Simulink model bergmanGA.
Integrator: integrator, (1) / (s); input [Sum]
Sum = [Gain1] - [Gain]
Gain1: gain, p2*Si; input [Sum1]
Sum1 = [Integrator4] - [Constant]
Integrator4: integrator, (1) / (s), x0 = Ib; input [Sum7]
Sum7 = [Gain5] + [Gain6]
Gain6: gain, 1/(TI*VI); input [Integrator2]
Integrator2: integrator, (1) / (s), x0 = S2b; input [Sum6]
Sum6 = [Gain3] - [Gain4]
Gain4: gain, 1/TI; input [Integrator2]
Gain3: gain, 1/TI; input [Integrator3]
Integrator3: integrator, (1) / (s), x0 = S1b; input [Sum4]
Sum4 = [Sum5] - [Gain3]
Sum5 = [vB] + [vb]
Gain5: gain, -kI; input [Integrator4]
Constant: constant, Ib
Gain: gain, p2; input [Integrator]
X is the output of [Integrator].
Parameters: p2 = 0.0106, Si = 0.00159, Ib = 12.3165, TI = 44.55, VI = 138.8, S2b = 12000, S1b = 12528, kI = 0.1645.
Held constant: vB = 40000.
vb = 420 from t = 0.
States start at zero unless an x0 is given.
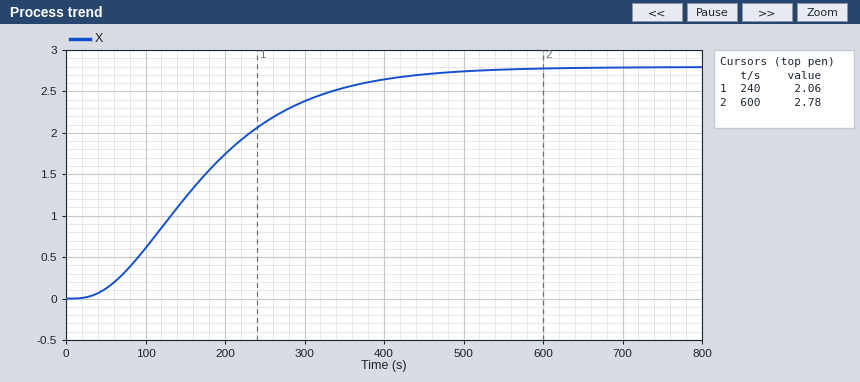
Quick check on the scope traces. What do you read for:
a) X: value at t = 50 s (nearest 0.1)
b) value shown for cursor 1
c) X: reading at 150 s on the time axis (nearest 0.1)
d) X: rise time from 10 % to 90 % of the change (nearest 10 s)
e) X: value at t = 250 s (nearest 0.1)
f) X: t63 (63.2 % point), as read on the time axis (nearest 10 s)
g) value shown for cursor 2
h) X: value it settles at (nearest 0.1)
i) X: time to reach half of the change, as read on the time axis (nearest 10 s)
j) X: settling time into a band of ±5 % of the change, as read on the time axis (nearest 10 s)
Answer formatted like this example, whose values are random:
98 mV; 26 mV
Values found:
0.1; 2.06; 1.2; 270 s; 2.1; 200 s; 2.78; 2.8; 170 s; 410 s
